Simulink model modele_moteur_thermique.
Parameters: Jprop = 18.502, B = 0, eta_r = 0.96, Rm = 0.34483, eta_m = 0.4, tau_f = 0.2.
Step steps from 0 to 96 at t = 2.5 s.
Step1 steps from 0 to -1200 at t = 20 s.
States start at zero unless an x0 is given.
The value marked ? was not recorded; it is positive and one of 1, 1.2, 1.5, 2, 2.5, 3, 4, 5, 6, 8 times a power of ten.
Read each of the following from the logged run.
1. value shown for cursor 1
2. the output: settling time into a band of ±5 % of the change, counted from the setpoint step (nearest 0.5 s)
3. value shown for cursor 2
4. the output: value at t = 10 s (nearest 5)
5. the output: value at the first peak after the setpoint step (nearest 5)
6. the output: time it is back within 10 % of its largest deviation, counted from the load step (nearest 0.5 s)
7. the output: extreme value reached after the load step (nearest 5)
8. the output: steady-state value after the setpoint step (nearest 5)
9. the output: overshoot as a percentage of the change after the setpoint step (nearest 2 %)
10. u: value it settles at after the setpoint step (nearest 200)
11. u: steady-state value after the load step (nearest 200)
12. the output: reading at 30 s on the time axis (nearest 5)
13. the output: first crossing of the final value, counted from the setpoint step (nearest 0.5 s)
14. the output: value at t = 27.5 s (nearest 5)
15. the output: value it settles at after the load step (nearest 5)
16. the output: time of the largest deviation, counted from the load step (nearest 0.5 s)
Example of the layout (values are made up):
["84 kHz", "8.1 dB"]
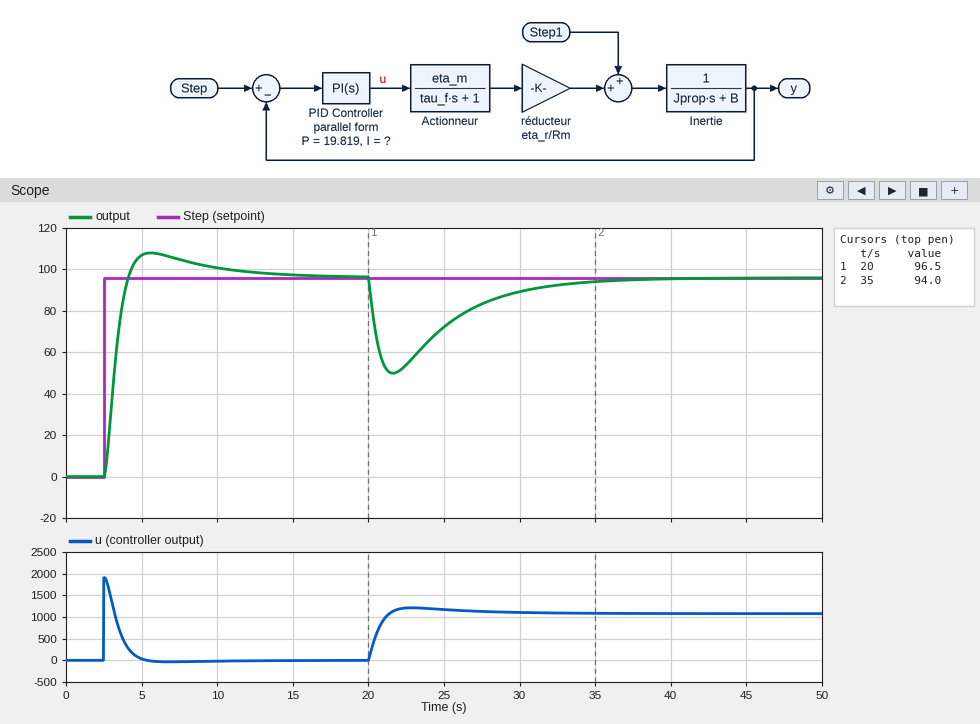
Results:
["96.5", "7.5 s", "94.0", "100", "110", "11.5 s", "50", "95", "12 %", "0", "1000", "90", "1.5 s", "85", "95", "1.5 s"]
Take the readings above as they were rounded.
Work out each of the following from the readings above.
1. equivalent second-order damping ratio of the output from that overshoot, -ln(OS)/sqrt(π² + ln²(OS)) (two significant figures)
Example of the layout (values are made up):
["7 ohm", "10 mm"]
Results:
["0.56"]
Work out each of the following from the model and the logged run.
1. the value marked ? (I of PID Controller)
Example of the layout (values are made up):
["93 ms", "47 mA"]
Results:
["4"]
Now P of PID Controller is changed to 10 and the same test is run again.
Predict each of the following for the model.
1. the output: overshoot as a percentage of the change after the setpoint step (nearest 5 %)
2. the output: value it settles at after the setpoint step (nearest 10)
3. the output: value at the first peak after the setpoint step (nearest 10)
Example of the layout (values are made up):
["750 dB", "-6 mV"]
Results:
["30 %", "100", "120"]
